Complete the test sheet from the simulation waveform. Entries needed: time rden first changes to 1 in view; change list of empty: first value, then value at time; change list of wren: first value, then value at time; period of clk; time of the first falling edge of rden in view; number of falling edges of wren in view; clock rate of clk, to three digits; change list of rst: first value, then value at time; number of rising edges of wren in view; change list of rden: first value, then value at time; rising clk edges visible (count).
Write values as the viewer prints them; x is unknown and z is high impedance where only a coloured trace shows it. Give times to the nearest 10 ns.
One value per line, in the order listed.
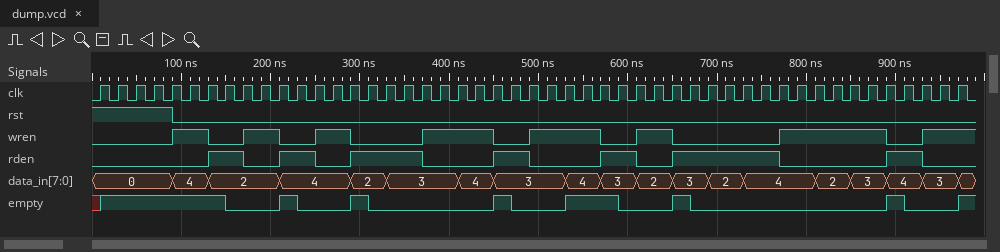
130 ns
x, 1 at 10 ns, 0 at 150 ns, 1 at 210 ns, 0 at 230 ns, 1 at 290 ns, 0 at 310 ns, 1 at 450 ns, 0 at 470 ns, 1 at 530 ns, 0 at 590 ns, 1 at 650 ns, 0 at 670 ns, 1 at 890 ns, 0 at 910 ns, 1 at 970 ns
0, 1 at 90 ns, 0 at 130 ns, 1 at 170 ns, 0 at 210 ns, 1 at 250 ns, 0 at 290 ns, 1 at 370 ns, 0 at 450 ns, 1 at 490 ns, 0 at 570 ns, 1 at 610 ns, 0 at 650 ns, 1 at 770 ns, 0 at 890 ns, 1 at 930 ns
20 ns
170 ns
7
50.0 MHz
1, 0 at 90 ns
8
0, 1 at 130 ns, 0 at 170 ns, 1 at 210 ns, 0 at 250 ns, 1 at 290 ns, 0 at 370 ns, 1 at 450 ns, 0 at 490 ns, 1 at 570 ns, 0 at 610 ns, 1 at 650 ns, 0 at 770 ns, 1 at 890 ns, 0 at 930 ns
49
